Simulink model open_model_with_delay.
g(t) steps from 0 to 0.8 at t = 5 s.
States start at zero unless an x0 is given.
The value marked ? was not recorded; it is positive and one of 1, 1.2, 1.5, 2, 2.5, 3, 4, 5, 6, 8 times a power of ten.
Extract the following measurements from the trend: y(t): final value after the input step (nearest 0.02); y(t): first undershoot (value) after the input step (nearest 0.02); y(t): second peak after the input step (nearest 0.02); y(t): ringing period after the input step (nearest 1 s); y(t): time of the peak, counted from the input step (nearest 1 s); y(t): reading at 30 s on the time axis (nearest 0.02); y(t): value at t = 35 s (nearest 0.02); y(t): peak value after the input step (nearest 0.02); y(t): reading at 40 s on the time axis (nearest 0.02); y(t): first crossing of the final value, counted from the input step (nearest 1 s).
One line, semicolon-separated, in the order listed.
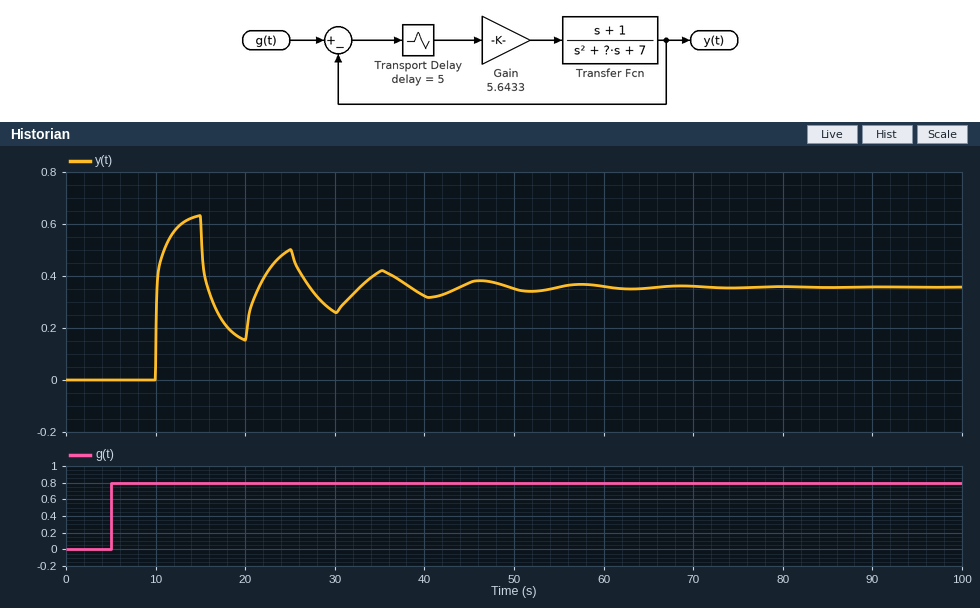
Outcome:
0.36; 0.16; 0.50; 10 s; 10 s; 0.26; 0.42; 0.64; 0.32; 5 s
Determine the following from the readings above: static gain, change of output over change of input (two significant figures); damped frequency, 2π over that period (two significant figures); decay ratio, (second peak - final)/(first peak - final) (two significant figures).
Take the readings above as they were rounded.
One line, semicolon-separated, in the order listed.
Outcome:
0.45; 0.63 rad/s; 0.50
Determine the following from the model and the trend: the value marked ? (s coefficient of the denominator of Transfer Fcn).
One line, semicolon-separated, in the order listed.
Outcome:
12
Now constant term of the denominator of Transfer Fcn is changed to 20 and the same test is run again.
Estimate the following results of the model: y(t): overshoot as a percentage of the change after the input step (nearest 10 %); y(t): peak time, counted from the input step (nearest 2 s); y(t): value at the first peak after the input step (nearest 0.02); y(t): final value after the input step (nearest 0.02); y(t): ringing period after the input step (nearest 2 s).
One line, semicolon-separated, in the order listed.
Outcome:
100 %; 6 s; 0.36; 0.18; 10 s
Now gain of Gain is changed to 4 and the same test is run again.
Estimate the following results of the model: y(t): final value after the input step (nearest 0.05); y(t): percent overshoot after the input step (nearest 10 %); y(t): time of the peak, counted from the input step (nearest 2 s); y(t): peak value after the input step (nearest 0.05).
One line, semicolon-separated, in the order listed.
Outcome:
0.30; 50 %; 10 s; 0.45
